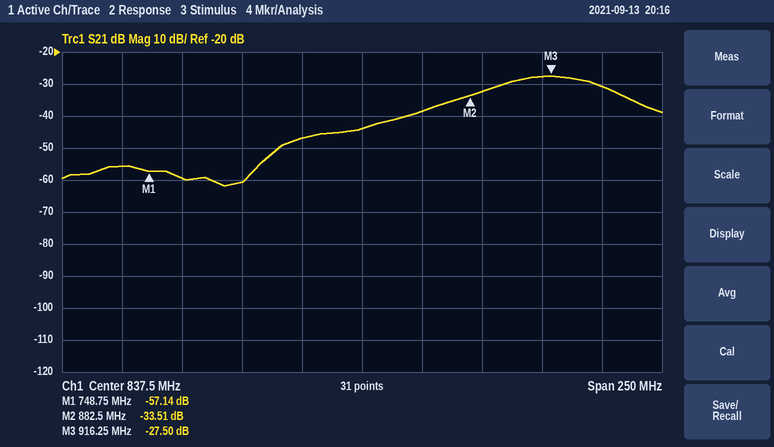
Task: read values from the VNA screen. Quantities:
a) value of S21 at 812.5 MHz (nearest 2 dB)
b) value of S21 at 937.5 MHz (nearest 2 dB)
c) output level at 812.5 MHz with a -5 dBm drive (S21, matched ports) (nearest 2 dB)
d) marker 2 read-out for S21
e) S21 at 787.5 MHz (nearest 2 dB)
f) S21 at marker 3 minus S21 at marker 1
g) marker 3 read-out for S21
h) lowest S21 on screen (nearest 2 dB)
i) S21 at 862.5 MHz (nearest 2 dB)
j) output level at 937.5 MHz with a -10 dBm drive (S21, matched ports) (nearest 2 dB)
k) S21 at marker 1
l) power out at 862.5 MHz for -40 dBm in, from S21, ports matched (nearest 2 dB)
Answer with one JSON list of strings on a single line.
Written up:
["-46 dB", "-30 dB", "-52 dBm", "-33.51 dB", "-60 dB", "29.64 dB", "-27.50 dB", "-62 dB", "-38 dB", "-40 dBm", "-57.14 dB", "-78 dBm"]
